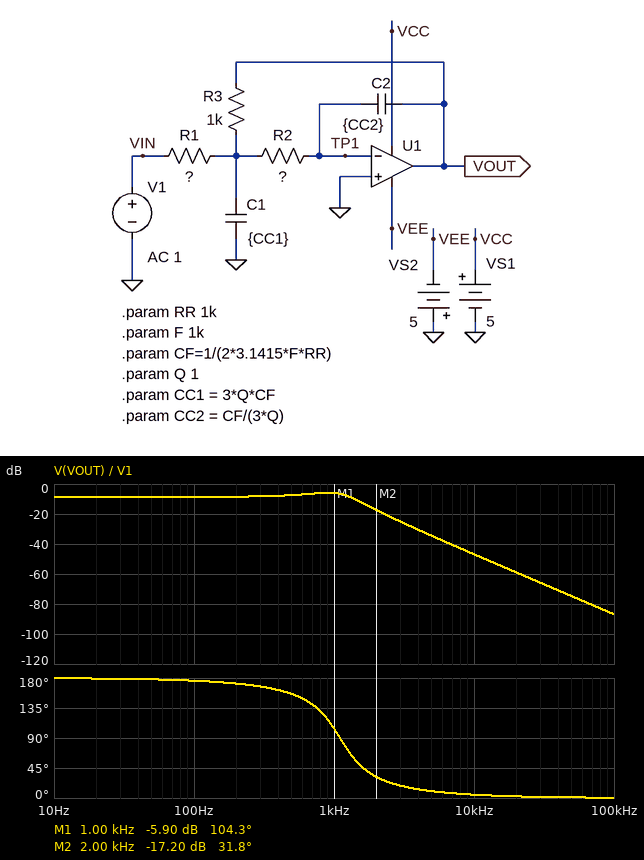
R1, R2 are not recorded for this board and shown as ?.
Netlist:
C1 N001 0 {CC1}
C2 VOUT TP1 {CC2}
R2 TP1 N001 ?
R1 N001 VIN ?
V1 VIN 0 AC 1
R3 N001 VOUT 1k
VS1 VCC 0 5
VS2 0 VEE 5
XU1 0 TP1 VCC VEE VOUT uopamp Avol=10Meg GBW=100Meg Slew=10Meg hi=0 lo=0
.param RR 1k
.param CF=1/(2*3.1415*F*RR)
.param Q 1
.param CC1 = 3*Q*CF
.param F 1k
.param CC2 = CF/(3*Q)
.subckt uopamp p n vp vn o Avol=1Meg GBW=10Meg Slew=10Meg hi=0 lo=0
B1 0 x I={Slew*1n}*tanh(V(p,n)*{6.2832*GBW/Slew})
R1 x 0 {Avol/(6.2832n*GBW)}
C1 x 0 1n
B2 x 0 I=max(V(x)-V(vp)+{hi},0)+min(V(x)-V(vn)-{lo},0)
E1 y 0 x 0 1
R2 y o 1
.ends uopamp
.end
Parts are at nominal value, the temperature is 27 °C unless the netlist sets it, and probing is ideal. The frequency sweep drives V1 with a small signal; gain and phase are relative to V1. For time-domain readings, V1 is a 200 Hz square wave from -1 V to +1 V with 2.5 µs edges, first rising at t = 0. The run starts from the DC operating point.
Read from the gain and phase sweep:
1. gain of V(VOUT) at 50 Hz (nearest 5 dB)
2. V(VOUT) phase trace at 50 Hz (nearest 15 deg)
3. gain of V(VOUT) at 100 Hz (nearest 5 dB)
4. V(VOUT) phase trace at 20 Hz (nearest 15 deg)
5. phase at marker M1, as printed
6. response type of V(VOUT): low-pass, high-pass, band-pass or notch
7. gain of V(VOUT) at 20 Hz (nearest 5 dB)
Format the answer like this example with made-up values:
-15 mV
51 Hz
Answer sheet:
-10 dB
180 deg
-10 dB
180 deg
104.3 deg
low-pass
-10 dB
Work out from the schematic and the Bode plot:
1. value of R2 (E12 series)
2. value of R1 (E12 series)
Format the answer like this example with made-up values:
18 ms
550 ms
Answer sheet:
820 Ω
2.7 kΩ
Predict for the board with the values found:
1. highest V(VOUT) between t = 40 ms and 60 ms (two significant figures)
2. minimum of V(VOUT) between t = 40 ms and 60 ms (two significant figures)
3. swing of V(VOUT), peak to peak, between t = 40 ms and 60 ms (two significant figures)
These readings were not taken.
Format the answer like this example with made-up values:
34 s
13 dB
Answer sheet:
570 mV
-570 mV
1.1 V
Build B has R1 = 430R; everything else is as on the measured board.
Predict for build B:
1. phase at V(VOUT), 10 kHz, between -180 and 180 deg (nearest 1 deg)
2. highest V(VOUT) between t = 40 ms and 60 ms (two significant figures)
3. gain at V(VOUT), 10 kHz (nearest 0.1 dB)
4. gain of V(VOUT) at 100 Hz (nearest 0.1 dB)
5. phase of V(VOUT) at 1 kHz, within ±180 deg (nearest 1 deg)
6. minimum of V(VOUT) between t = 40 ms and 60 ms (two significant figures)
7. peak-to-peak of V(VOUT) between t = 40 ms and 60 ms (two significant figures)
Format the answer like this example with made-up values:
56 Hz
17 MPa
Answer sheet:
9 deg
2.6 V
-30.9 dB
7.3 dB
98 deg
-2.6 V
5.1 V
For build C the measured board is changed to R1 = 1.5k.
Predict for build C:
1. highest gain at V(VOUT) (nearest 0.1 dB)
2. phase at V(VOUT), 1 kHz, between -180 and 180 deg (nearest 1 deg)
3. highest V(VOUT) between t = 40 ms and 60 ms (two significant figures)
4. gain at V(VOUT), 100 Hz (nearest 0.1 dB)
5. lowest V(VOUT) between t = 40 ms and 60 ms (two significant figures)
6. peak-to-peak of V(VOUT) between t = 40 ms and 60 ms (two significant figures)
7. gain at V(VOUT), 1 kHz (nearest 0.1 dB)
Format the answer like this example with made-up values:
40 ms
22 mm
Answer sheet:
-1.4 dB
103 deg
960 mV
-3.5 dB
-960 mV
1.9 V
-1.7 dB
